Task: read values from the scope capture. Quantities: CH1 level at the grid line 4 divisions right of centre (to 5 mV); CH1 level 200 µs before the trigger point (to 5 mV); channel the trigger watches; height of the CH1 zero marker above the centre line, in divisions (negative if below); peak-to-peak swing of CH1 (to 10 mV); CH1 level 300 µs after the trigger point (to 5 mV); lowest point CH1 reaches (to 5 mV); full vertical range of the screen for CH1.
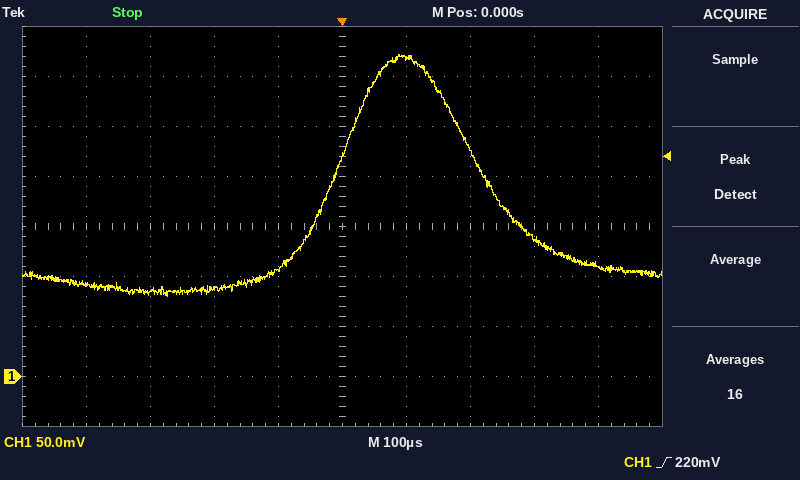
110 mV
90 mV
CH1
-3.0 div
240 mV
140 mV
80 mV
400 mV
